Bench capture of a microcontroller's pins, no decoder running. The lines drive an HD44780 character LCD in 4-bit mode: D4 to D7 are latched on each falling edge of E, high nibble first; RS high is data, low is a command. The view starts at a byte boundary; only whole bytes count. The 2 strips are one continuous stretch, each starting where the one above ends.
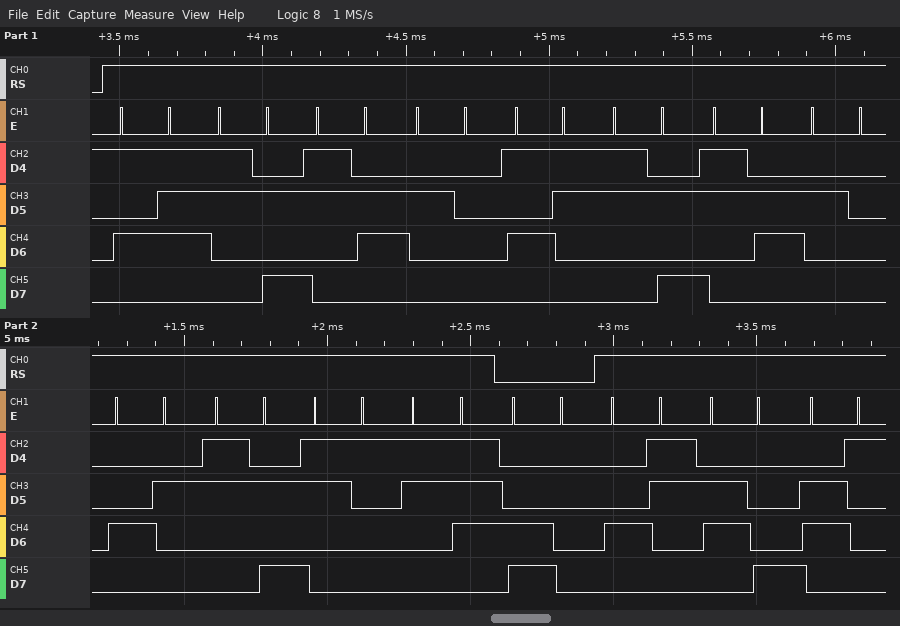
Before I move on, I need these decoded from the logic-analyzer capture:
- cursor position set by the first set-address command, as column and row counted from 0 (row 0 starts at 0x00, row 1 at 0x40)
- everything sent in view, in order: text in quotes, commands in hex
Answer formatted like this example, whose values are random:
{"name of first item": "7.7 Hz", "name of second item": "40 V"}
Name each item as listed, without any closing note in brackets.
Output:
{"cursor position set by the first set-address command, as column and row counted from 0": "column 0, row 1", "everything sent in view, in order: text in quotes, commands in hex": "\"W:6 S:6 B:17\" 0xC0 \"Cha\""}
